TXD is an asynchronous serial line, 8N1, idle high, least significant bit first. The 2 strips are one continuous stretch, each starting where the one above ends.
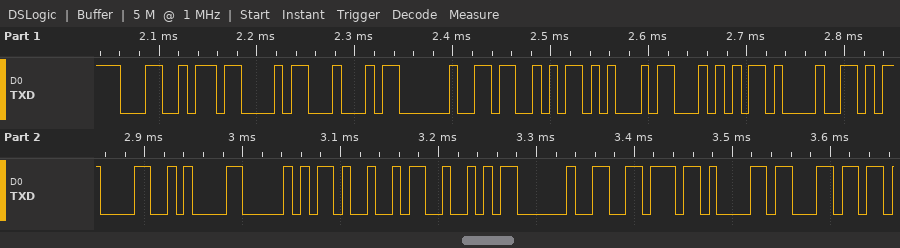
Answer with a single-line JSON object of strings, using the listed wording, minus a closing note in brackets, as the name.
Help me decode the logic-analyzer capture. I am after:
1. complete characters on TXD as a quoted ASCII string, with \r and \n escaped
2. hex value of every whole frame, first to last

{"complete characters on TXD as a quoted ASCII string, with \\r and \\n escaped": "\"LCD SET!\\r\\nPIR val\"", "hex value of every whole frame, first to last": "4C 43 44 20 53 45 54 21 0D 0A 50 49 52 20 76 61 6C"}
